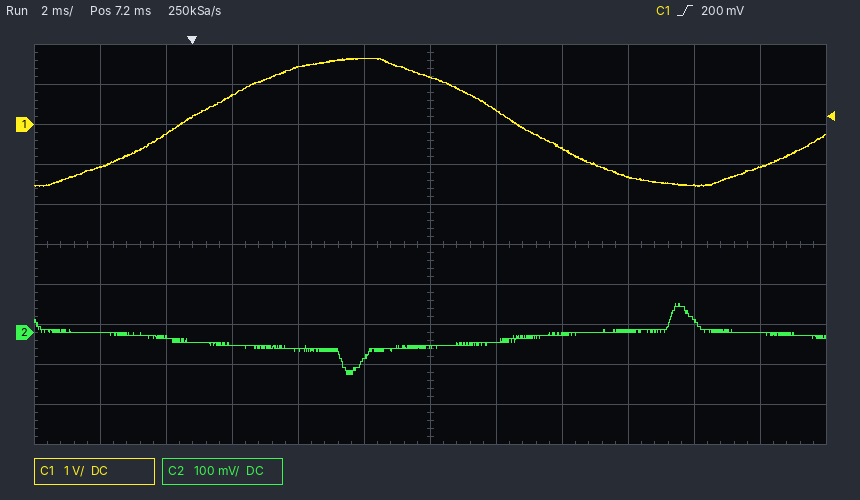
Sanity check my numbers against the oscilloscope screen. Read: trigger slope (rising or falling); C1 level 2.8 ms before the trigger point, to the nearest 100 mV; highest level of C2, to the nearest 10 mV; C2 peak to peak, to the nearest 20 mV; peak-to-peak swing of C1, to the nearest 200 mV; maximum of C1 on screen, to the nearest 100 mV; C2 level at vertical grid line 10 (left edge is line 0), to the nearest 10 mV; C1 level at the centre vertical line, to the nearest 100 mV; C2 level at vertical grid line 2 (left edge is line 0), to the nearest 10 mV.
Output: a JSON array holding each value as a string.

["rising", "-1.1 V", "70 mV", "180 mV", "3.2 V", "1.7 V", "30 mV", "1.2 V", "-10 mV"]
